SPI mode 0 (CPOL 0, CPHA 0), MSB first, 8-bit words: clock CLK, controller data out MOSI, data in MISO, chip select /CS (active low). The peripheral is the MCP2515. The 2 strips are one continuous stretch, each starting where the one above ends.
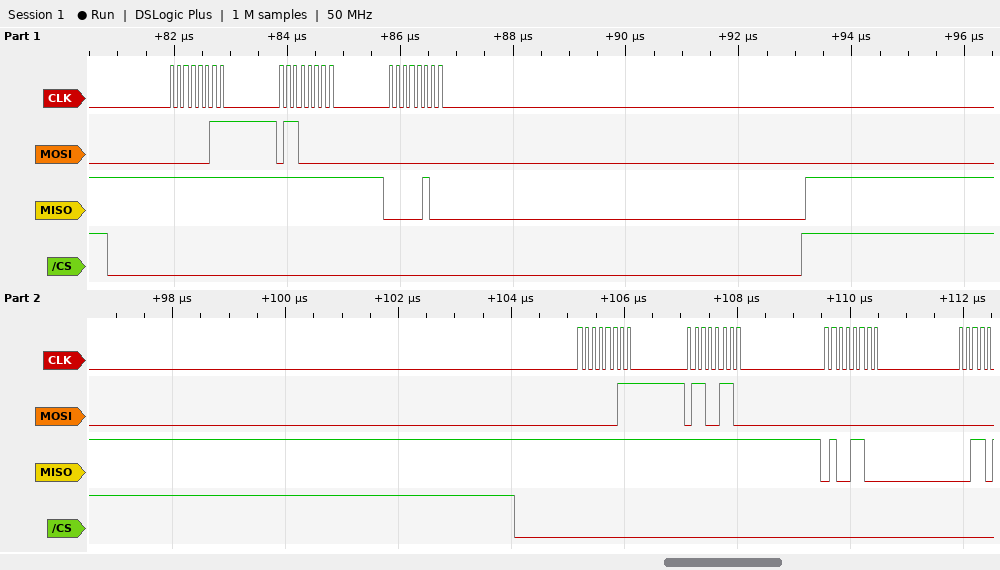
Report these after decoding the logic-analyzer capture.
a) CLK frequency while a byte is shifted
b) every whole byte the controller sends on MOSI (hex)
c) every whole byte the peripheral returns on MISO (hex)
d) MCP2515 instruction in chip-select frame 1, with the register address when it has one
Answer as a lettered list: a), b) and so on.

a) 8 MHz
b) 03 60 00 03 66 00
c) FF FF 04 FF FF 4C
d) READ 0x60
